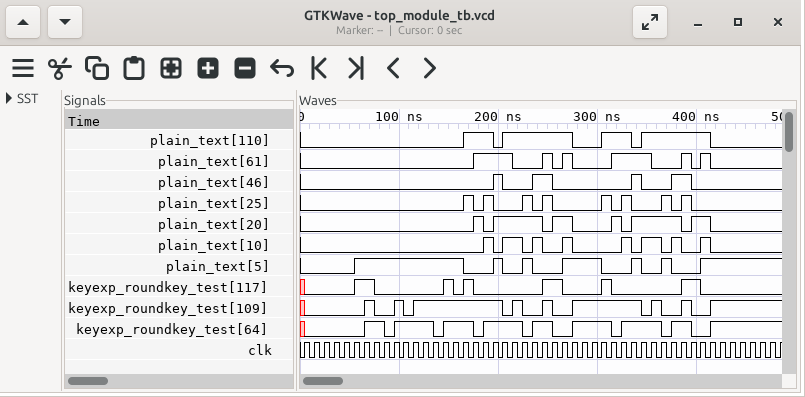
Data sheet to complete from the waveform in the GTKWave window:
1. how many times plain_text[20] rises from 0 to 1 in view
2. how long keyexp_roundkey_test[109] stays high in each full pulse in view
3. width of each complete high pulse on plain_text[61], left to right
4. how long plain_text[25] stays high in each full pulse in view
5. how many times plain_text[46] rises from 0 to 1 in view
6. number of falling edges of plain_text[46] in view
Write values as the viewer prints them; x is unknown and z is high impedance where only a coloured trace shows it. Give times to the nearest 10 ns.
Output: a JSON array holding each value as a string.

["6", "10 ns, 10 ns, 90 ns, 10 ns, 10 ns, 70 ns, 10 ns, 10 ns", "40 ns, 10 ns, 10 ns, 40 ns, 10 ns, 10 ns", "10 ns, 10 ns, 10 ns, 10 ns, 10 ns, 10 ns, 10 ns, 10 ns", "4", "4"]
